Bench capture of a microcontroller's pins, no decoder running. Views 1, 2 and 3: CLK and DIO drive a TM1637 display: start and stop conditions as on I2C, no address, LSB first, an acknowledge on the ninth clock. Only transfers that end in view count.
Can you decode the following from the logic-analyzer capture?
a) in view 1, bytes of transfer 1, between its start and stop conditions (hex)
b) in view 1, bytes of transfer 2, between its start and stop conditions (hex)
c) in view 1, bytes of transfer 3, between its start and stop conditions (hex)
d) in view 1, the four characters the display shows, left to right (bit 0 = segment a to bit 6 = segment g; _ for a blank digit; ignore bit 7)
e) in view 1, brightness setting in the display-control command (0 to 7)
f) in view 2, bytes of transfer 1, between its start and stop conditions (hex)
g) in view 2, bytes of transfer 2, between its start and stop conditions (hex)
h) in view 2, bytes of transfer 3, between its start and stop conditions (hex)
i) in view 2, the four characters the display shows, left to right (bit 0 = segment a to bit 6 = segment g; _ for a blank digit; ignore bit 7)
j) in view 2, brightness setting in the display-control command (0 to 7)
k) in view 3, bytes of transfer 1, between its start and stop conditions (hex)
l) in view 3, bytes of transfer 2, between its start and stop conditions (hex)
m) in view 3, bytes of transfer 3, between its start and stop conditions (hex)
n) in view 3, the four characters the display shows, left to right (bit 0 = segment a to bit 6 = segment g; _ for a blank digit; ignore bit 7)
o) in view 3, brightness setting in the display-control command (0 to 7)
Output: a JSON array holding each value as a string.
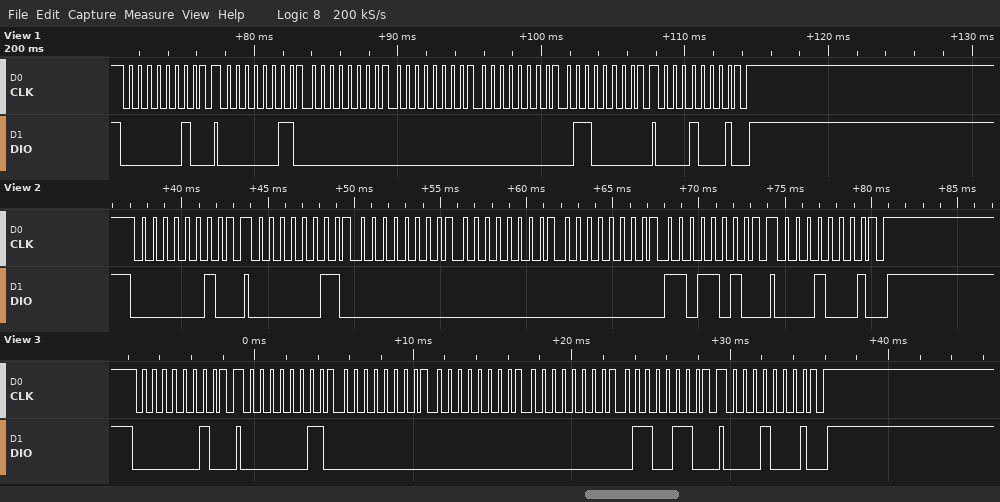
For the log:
["40", "C0 00 00 00 06", "88", "___1", "0", "40", "C0 00 00 00 5B", "88", "___2", "0", "40", "C0 00 00 00 66", "88", "___4", "0"]
